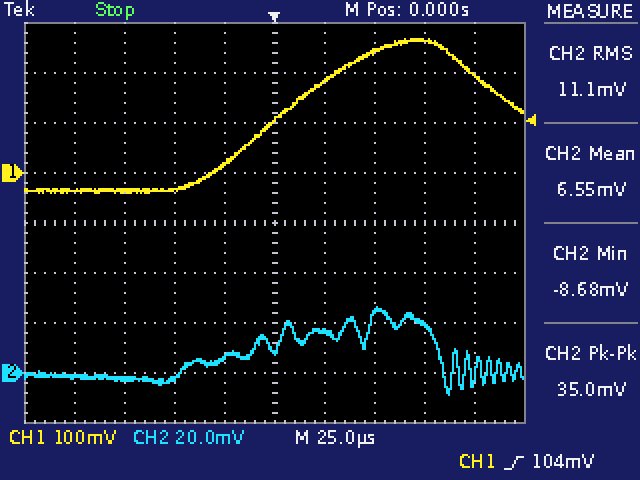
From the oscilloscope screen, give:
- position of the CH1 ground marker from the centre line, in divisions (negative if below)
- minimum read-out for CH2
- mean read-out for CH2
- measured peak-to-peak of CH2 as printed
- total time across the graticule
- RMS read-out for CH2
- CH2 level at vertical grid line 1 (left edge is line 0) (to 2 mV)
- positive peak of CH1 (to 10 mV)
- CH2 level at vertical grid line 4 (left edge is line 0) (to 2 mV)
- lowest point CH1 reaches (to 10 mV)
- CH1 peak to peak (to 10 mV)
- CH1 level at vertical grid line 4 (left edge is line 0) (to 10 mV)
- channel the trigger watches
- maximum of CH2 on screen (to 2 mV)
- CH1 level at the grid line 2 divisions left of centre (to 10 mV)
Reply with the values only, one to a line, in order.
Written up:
+1.0 div
-8.68 mV
6.55 mV
35.0 mV
250 µs
11.1 mV
-2 mV
270 mV
6 mV
-40 mV
310 mV
20 mV
CH1
26 mV
-30 mV
